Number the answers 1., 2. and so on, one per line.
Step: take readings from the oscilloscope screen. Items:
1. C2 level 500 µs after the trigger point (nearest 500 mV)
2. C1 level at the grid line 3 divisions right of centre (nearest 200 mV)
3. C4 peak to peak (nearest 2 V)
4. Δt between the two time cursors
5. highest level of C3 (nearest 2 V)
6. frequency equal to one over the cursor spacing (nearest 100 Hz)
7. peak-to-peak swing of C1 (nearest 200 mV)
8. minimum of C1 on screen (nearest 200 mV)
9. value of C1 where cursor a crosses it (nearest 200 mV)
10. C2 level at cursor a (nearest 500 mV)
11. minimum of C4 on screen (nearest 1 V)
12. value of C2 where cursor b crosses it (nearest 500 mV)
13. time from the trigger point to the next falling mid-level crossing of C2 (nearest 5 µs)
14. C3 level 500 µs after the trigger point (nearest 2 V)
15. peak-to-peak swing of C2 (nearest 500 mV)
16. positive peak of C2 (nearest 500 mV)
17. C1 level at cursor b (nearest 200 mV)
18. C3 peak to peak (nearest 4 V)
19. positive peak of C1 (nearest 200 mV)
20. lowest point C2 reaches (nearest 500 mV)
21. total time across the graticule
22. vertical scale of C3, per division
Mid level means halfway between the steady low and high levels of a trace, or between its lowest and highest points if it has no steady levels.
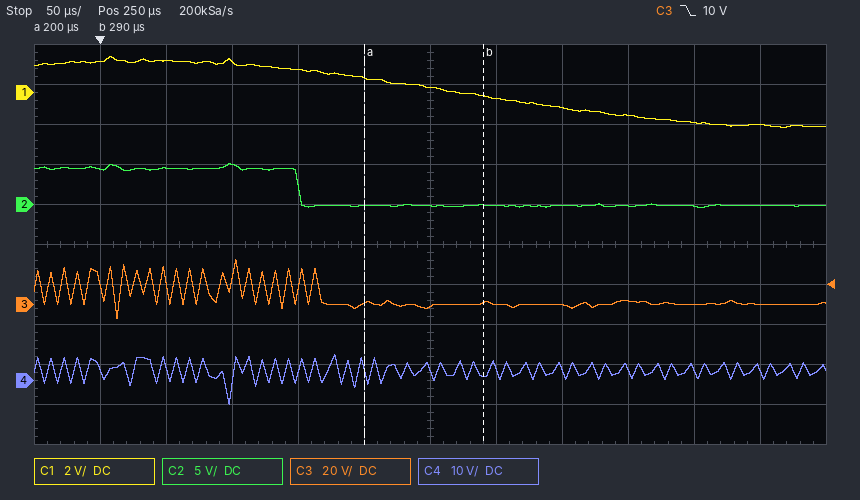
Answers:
1. 0.0 V
2. -1.2 V
3. 12 V
4. 90 µs
5. 22 V
6. 11.1 kHz
7. 3.6 V
8. -1.8 V
9. 800 mV
10. 0.0 V
11. -6 V
12. 0.0 V
13. 150 µs
14. 0 V
15. 5.5 V
16. 5.0 V
17. -200 mV
18. 28 V
19. 1.8 V
20. -500 mV
21. 600 µs
22. 20 V
